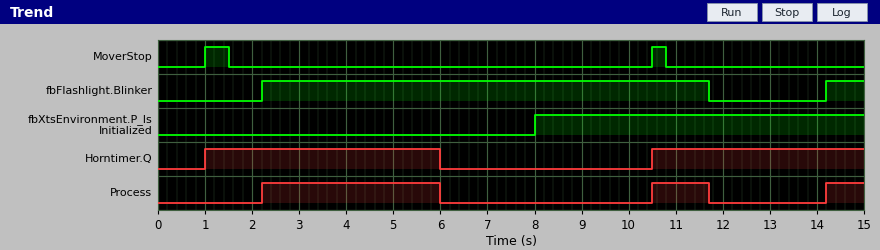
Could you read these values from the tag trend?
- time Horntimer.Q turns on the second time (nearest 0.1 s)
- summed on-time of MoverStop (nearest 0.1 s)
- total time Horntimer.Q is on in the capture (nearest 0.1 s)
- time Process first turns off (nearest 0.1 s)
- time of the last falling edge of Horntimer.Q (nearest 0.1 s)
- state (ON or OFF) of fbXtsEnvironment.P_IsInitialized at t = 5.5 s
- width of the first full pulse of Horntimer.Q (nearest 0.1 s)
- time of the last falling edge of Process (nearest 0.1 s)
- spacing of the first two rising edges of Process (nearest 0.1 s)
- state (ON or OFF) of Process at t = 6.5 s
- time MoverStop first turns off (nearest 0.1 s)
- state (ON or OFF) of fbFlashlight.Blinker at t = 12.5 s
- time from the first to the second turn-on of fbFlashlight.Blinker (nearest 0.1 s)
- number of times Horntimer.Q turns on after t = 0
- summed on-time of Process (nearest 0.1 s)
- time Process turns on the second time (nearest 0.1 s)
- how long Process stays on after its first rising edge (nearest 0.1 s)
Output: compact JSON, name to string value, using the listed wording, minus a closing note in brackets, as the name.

{"time Horntimer.Q turns on the second time": "10.5 s", "summed on-time of MoverStop": "0.8 s", "total time Horntimer.Q is on in the capture": "9.5 s", "time Process first turns off": "6.0 s", "time of the last falling edge of Horntimer.Q": "6.0 s", "state (ON or OFF) of fbXtsEnvironment.P_IsInitialized at t = 5.5 s": "OFF", "width of the first full pulse of Horntimer.Q": "5.0 s", "time of the last falling edge of Process": "11.7 s", "spacing of the first two rising edges of Process": "8.3 s", "state (ON or OFF) of Process at t = 6.5 s": "OFF", "time MoverStop first turns off": "1.5 s", "state (ON or OFF) of fbFlashlight.Blinker at t = 12.5 s": "OFF", "time from the first to the second turn-on of fbFlashlight.Blinker": "12.0 s", "number of times Horntimer.Q turns on after t = 0": "2", "summed on-time of Process": "5.8 s", "time Process turns on the second time": "10.5 s", "how long Process stays on after its first rising edge": "3.8 s"}
